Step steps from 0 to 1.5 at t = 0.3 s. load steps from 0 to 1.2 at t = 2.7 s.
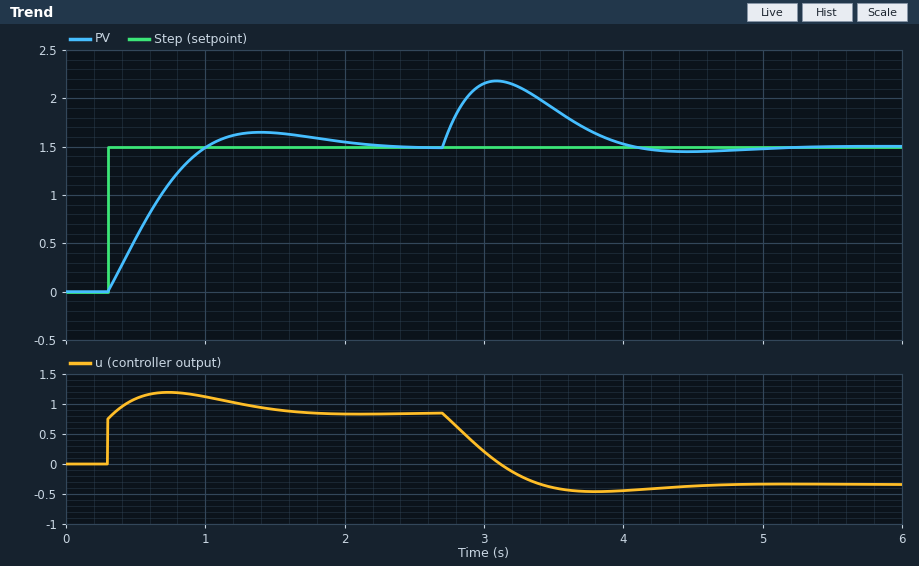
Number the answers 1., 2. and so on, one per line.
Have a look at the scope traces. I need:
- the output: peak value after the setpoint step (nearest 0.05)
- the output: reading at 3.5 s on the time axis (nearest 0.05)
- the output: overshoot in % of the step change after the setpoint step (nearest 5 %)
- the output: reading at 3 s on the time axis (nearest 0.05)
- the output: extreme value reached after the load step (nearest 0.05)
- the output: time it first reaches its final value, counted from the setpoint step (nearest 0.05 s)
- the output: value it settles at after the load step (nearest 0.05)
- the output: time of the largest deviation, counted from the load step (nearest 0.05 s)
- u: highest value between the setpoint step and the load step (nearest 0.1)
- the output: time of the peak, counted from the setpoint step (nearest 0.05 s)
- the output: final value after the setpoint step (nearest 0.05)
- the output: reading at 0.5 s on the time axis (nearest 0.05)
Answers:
1. 1.65
2. 1.90
3. 10 %
4. 2.15
5. 2.20
6. 0.70 s
7. 1.50
8. 0.40 s
9. 1.2
10. 1.10 s
11. 1.50
12. 0.55
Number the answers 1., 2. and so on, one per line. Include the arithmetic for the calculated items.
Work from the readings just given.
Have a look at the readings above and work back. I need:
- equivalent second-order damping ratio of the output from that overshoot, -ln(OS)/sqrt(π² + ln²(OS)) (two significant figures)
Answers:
1. ln(0.1) = -2.303; 2.303 / sqrt(9.870 + 5.302) = 0.59
